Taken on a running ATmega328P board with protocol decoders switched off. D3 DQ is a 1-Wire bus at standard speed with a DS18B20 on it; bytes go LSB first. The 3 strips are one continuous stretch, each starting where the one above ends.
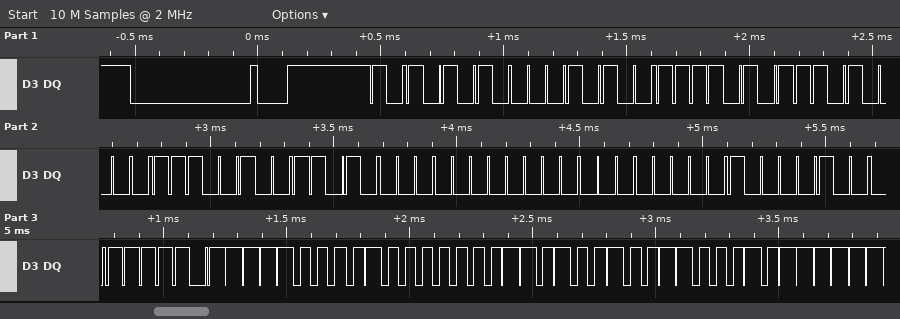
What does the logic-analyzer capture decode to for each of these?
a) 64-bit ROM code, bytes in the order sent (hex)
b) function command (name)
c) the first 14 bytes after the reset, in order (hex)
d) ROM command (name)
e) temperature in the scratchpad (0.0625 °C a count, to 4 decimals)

28 AF 0B 27 0B 00 00 21
Read Scratchpad
55 28 AF 0B 27 0B 00 00 21 BE 0F 01 4B 46
Match ROM
16.9375 °C
